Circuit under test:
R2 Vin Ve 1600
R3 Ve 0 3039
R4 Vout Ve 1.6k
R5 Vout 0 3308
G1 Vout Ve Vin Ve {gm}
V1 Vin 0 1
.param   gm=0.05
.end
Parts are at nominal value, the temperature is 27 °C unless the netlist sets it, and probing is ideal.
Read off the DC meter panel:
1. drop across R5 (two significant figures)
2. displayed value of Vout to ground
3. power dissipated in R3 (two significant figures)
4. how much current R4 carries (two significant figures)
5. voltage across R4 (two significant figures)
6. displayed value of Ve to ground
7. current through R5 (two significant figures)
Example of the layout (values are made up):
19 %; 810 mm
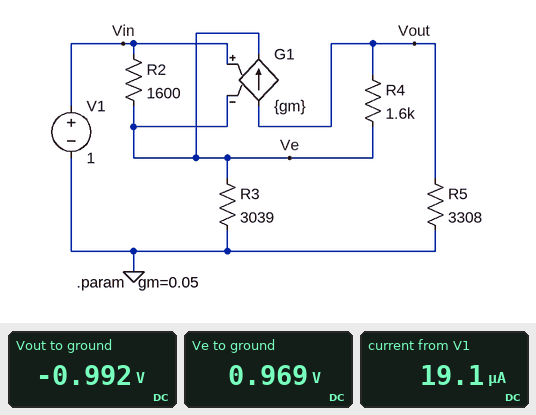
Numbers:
990 mV; -0.992 V; 310 µW; 1.2 mA; 2.0 V; 0.969 V; 300 µA
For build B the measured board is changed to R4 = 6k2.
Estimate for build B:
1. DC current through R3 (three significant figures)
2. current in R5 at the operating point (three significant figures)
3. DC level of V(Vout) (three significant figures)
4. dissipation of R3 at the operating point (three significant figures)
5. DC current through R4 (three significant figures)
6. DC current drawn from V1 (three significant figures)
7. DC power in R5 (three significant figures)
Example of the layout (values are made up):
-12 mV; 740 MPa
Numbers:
325 µA; 317 µA; -1.05 V; 321 µW; 328 µA; 8.06 µA; 332 µW
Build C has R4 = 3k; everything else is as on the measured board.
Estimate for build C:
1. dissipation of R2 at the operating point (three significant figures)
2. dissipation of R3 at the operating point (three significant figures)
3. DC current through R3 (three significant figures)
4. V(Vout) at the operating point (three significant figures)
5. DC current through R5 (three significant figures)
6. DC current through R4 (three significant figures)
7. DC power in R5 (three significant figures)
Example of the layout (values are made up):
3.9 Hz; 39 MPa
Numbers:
240 nW; 316 µW; 323 µA; -1.03 V; 310 µA; 669 µA; 319 µW
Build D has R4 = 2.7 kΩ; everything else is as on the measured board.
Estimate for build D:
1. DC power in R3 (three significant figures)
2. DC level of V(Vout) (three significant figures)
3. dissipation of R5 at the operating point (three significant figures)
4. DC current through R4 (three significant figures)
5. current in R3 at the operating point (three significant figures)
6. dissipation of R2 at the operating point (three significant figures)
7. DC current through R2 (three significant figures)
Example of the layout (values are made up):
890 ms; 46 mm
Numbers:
315 µW; -1.02 V; 316 µW; 741 µA; 322 µA; 276 nW; 13.1 µA
